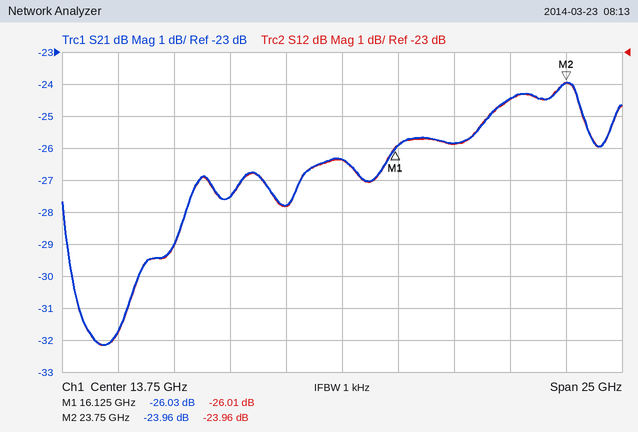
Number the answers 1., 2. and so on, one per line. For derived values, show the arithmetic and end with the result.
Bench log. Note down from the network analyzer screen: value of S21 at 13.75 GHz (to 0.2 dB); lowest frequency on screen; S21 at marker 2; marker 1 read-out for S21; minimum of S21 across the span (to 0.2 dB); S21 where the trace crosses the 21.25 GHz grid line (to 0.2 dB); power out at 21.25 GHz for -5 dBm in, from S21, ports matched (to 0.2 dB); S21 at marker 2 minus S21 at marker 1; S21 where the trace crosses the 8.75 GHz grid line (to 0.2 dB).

1. -26.4 dB
2. 1.25 GHz
3. -23.96 dB
4. -26.03 dB
5. -32.2 dB
6. -24.4 dB
7. -5 dBm + (-24.4 dB) = -29.4 dBm
8. -23.96 − (-26.03) = 2.07 dB
9. -27.6 dB
